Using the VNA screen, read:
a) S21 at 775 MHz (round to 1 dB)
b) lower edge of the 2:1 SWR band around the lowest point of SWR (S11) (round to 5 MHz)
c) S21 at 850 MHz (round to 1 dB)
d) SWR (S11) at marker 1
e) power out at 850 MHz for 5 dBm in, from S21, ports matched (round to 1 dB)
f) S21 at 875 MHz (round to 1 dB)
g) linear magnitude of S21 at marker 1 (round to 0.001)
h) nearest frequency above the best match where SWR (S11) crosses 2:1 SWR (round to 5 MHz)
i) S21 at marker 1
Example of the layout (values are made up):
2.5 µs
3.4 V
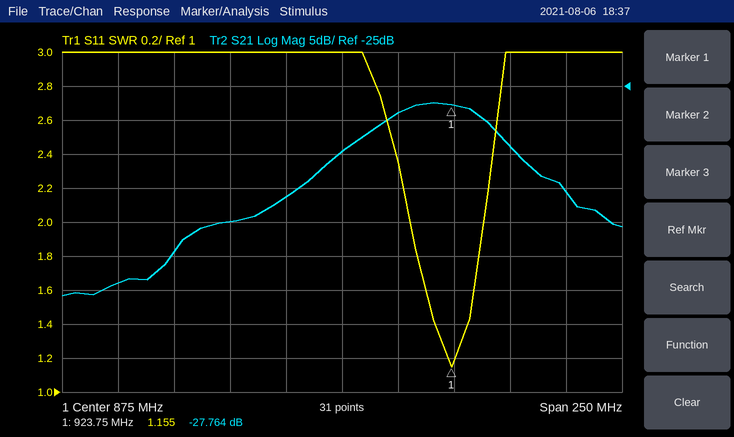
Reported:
-54 dB
905 MHz
-41 dB
1.155
-36 dBm
-35 dB
0.041
940 MHz
-27.764 dB
